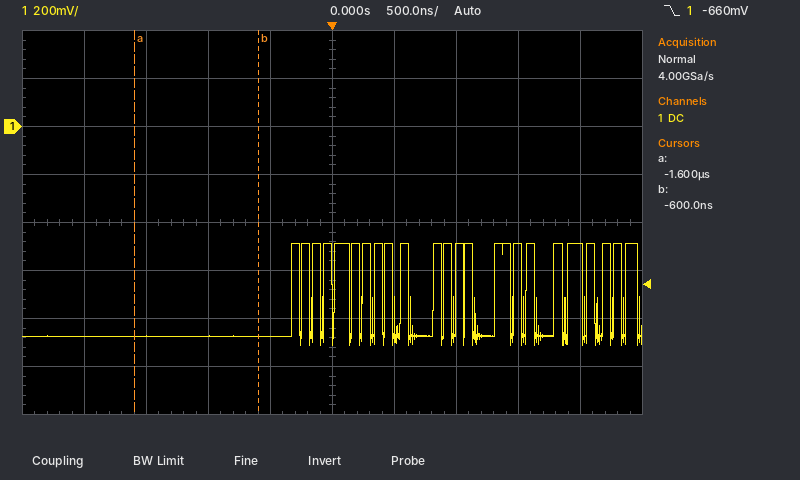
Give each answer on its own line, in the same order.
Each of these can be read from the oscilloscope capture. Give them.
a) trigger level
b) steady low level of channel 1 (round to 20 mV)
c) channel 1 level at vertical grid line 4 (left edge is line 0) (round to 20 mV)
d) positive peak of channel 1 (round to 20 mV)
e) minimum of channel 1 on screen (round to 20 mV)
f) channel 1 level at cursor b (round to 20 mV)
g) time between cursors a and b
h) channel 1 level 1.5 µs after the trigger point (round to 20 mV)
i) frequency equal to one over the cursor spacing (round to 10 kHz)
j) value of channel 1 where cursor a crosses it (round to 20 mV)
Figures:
-660 mV
-880 mV
-880 mV
-480 mV
-920 mV
-880 mV
1.00 µs
-480 mV
1.00 MHz
-880 mV
